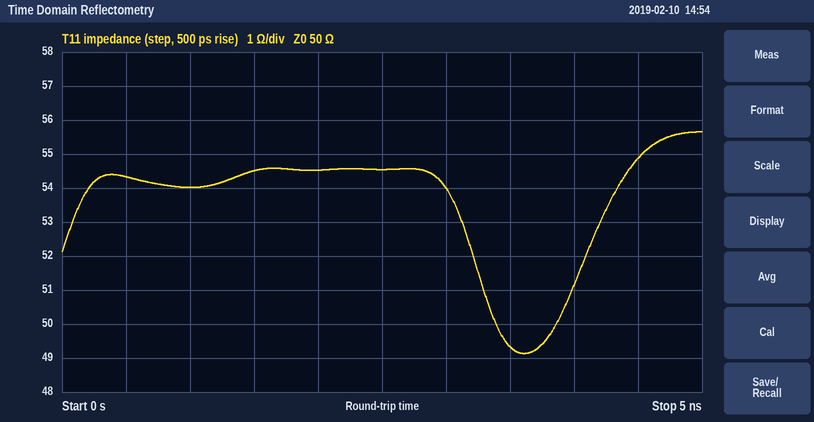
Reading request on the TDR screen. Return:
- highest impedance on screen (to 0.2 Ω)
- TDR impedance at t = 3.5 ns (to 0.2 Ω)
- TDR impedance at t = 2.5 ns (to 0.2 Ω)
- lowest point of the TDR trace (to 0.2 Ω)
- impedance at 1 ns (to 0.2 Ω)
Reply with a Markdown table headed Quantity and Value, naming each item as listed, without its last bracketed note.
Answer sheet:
| Quantity | Value |
|---|---|
| highest impedance on screen | 55.6 Ω |
| TDR impedance at t = 3.5 ns | 49.4 Ω |
| TDR impedance at t = 2.5 ns | 54.6 Ω |
| lowest point of the TDR trace | 49.2 Ω |
| impedance at 1 ns | 54.0 Ω |
